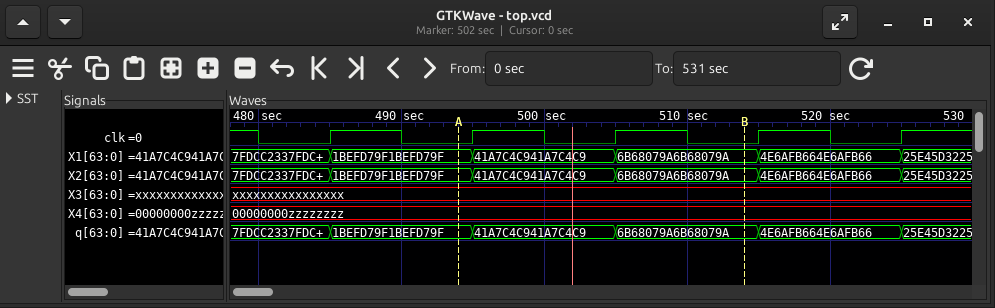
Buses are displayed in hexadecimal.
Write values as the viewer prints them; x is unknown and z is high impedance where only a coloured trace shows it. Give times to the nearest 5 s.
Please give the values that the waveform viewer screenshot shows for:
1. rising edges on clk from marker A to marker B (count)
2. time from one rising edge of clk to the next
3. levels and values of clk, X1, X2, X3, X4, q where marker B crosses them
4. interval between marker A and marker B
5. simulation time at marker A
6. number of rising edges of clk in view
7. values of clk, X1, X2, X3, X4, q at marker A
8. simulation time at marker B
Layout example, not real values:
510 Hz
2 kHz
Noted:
2
10 s
clk=0, X1=6B68079A6B68079A, X2=6B68079A6B68079A, X3=xxxxxxxxxxxxxxxx, X4=00000000zzzzzzzz, q=6B68079A6B68079A
20 s
495 s
5
clk=0, X1=1BEFD79F1BEFD79F, X2=1BEFD79F1BEFD79F, X3=xxxxxxxxxxxxxxxx, X4=00000000zzzzzzzz, q=1BEFD79F1BEFD79F
515 s
